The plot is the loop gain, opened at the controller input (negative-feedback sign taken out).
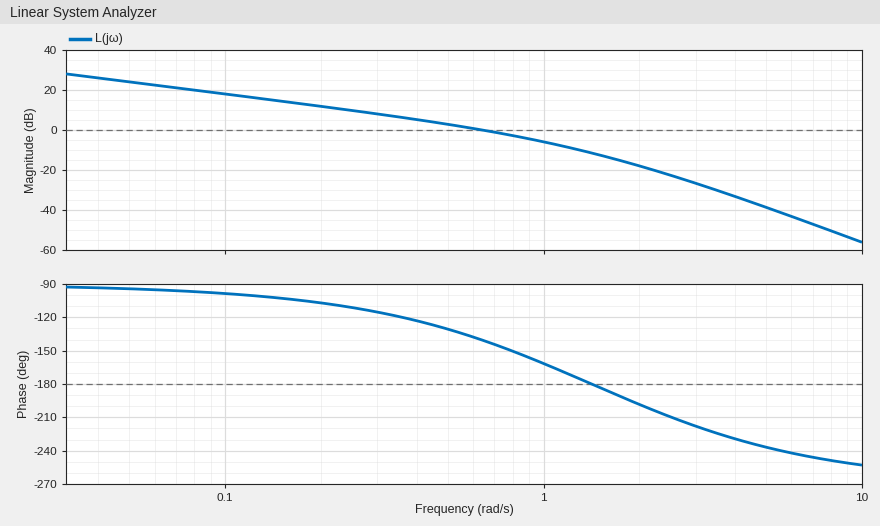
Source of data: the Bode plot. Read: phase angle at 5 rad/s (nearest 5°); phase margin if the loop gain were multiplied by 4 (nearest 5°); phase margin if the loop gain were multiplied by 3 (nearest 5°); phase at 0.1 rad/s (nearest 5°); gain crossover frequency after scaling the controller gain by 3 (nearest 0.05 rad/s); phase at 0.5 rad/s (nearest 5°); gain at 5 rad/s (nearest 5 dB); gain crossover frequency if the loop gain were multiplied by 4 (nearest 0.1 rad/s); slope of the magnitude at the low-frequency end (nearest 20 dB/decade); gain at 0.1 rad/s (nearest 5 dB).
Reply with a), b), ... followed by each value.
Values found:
a) -235°
b) 0°
c) 5°
d) -100°
e) 1.25 rad/s
f) -130°
g) -40 dB
h) 1.5 rad/s
i) -20 dB/decade
j) 20 dB
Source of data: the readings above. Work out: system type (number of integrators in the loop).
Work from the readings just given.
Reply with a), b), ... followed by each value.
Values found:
a) 1
